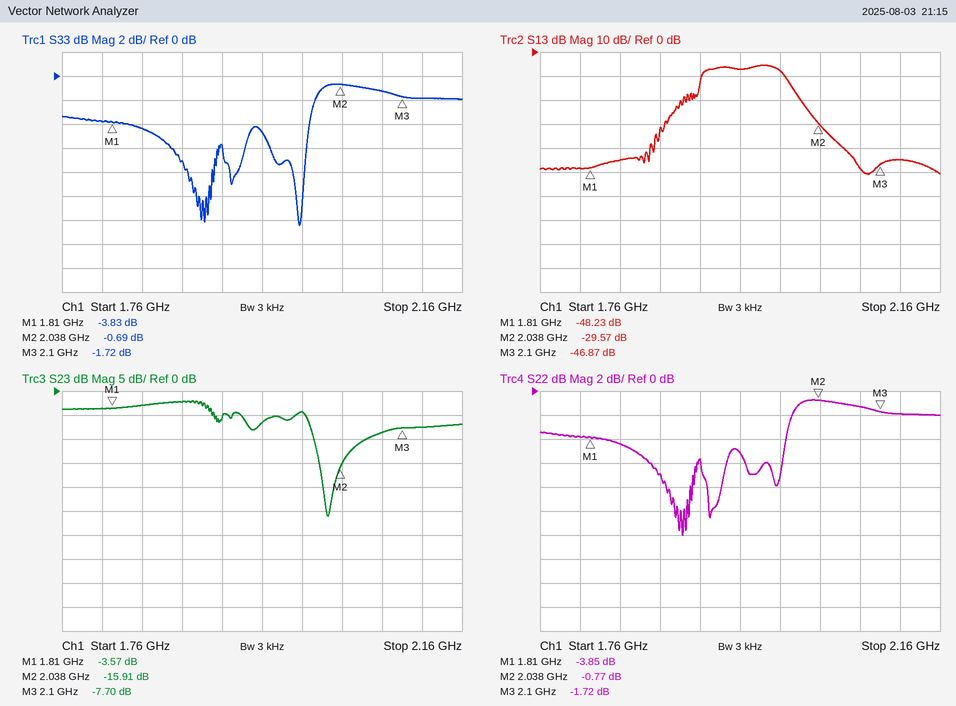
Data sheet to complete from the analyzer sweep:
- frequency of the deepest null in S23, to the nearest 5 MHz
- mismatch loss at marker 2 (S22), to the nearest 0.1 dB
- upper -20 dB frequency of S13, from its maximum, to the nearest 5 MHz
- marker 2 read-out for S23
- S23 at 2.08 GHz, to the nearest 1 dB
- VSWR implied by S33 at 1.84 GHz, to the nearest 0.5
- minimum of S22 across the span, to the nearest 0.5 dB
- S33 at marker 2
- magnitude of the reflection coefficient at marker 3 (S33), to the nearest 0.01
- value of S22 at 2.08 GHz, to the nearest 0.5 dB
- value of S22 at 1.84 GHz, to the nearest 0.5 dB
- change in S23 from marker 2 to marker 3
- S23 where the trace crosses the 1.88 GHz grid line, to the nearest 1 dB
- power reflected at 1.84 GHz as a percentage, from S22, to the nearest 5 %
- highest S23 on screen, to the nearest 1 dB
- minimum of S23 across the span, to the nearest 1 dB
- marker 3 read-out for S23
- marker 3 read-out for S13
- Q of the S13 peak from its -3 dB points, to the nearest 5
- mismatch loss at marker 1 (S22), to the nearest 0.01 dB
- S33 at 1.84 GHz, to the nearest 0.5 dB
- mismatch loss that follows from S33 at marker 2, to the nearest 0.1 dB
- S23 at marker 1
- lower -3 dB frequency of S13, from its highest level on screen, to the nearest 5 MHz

2.025 GHz
7.9 dB
2.030 GHz
-15.91 dB
-9 dB
4.0
-12.0 dB
-0.69 dB
0.82
-1.5 dB
-4.5 dB
8.21 dB
-2 dB
35 %
-2 dB
-26 dB
-7.70 dB
-46.87 dB
25
2.31 dB
-4.5 dB
8.3 dB
-3.57 dB
1.925 GHz
